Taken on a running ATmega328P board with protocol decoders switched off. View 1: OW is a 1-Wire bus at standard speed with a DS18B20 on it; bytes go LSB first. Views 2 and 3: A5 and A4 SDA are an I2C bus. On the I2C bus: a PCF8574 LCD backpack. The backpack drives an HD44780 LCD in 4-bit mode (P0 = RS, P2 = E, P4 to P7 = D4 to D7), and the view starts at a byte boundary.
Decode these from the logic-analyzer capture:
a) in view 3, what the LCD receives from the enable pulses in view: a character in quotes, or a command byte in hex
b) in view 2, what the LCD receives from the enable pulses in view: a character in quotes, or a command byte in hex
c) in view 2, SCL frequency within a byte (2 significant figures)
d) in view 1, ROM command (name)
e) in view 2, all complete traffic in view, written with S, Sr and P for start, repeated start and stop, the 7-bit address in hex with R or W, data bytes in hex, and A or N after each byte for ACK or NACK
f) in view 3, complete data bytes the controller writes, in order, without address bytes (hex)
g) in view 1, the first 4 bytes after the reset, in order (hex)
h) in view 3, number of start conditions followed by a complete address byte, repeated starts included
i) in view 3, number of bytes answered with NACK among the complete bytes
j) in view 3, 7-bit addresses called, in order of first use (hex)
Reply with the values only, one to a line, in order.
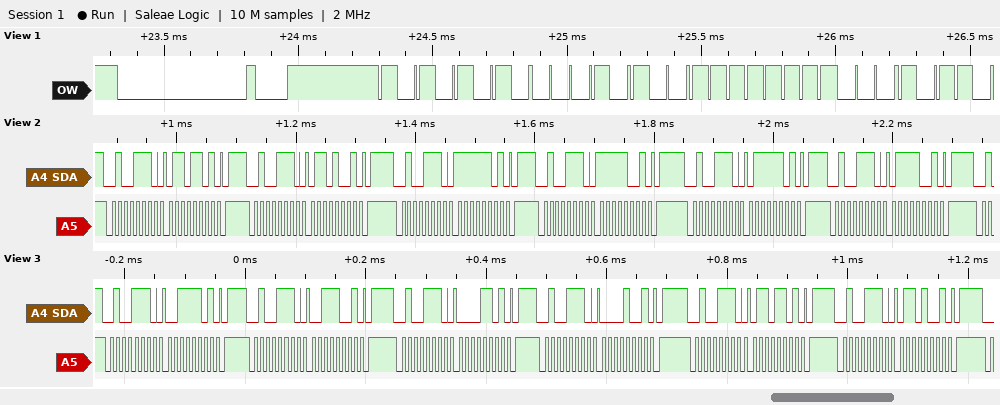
'0'
'o'
100 kHz
Match ROM
S 27W A 6D A P S 27W A 69 A P S 27W A FD A P S 27W A F9 A P S 27W A 7D A P S 27W A 79 A P
3D 39 0D 09 6D 69
55 28 FF 68
6
0
0x27
